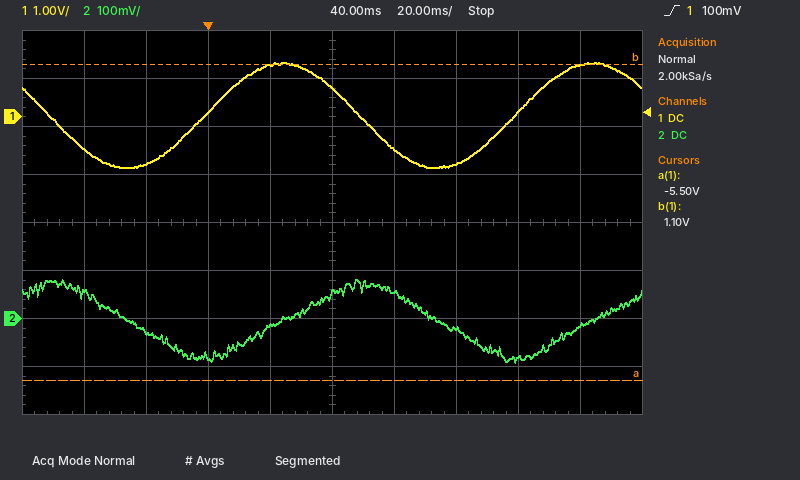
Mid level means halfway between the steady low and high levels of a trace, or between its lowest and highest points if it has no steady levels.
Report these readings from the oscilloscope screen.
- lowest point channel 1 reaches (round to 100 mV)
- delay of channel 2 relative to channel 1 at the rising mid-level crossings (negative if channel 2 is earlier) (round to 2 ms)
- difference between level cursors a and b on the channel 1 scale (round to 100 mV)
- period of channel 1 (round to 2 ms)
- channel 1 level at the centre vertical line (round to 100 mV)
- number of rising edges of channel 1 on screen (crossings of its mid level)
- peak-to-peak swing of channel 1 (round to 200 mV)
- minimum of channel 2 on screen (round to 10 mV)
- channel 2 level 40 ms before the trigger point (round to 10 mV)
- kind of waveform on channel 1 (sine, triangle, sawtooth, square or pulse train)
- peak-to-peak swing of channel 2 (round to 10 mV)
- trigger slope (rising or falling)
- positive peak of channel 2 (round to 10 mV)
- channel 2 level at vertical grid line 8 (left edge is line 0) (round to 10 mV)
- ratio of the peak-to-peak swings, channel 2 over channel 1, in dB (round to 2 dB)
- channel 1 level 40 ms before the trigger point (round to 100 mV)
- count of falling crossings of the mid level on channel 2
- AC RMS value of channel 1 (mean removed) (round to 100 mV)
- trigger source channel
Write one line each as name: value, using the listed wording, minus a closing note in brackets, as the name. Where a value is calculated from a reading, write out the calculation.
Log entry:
lowest point channel 1 reaches: -1.1 V
delay of channel 2 relative to channel 1 at the rising mid-level crossings (negative if channel 2 is earlier): +24 ms
difference between level cursors a and b on the channel 1 scale: 6.6 V
period of channel 1: 100 ms
channel 1 level at the centre vertical line: 600 mV
number of rising edges of channel 1 on screen: 2
peak-to-peak swing of channel 1: 2.2 V
minimum of channel 2 on screen: -90 mV
channel 2 level 40 ms before the trigger point: 50 mV
kind of waveform on channel 1: sine
peak-to-peak swing of channel 2: 80 mV − (-90 mV) = 170 mV
trigger slope: rising
positive peak of channel 2: 80 mV
channel 2 level at vertical grid line 8 (left edge is line 0): -80 mV
ratio of the peak-to-peak swings, channel 2 over channel 1, in dB: 20 log10(170 mV / 2.2 V) ≈ -22 dB
channel 1 level 40 ms before the trigger point: -700 mV
count of falling crossings of the mid level on channel 2: 2
AC RMS value of channel 1 (mean removed): 2.2 V / (2√2) ≈ 778 mV, so 800 mV to the nearest 100 mV
trigger source channel: channel 1
